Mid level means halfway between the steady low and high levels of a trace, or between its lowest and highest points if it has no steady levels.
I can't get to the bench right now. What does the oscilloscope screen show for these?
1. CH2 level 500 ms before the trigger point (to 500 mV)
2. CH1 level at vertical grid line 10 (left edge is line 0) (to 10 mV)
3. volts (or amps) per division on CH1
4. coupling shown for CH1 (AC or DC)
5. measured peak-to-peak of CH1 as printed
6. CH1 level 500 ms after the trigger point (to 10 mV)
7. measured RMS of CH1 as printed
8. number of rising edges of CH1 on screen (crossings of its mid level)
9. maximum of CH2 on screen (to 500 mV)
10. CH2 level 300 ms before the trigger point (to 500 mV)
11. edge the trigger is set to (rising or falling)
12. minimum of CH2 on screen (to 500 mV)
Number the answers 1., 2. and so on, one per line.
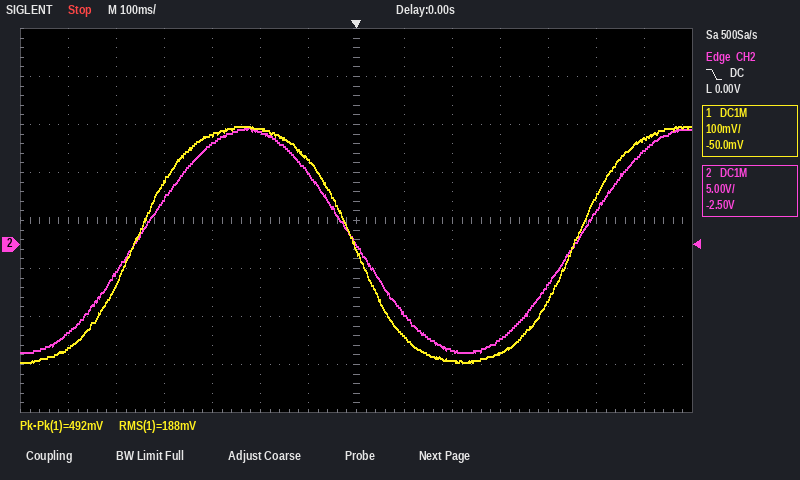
1. -3.0 V
2. -230 mV
3. 100 mV
4. DC
5. 492 mV
6. 100 mV
7. 188 mV
8. 2
9. 12.0 V
10. 10.5 V
11. falling
12. -11.0 V
